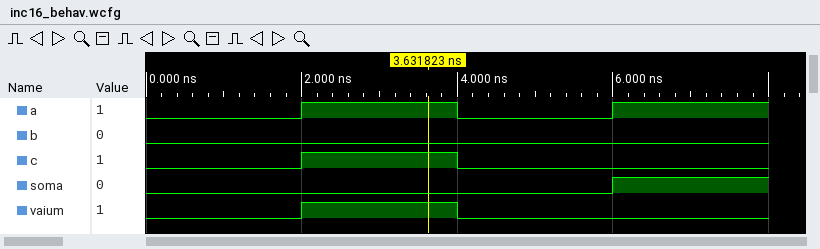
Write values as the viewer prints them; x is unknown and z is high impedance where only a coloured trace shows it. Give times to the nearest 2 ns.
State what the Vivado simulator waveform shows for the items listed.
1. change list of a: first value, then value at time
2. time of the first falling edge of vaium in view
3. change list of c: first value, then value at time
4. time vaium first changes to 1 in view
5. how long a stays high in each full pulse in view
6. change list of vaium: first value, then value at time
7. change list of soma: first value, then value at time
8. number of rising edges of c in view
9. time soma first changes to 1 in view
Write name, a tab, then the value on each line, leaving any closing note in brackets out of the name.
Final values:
change list of a: first value, then value at time	0, 1 at 2 ns, 0 at 4 ns, 1 at 6 ns
time of the first falling edge of vaium in view	4 ns
change list of c: first value, then value at time	0, 1 at 2 ns, 0 at 4 ns
time vaium first changes to 1 in view	2 ns
how long a stays high in each full pulse in view	2 ns
change list of vaium: first value, then value at time	0, 1 at 2 ns, 0 at 4 ns
change list of soma: first value, then value at time	0, 1 at 6 ns
number of rising edges of c in view	1
time soma first changes to 1 in view	6 ns
